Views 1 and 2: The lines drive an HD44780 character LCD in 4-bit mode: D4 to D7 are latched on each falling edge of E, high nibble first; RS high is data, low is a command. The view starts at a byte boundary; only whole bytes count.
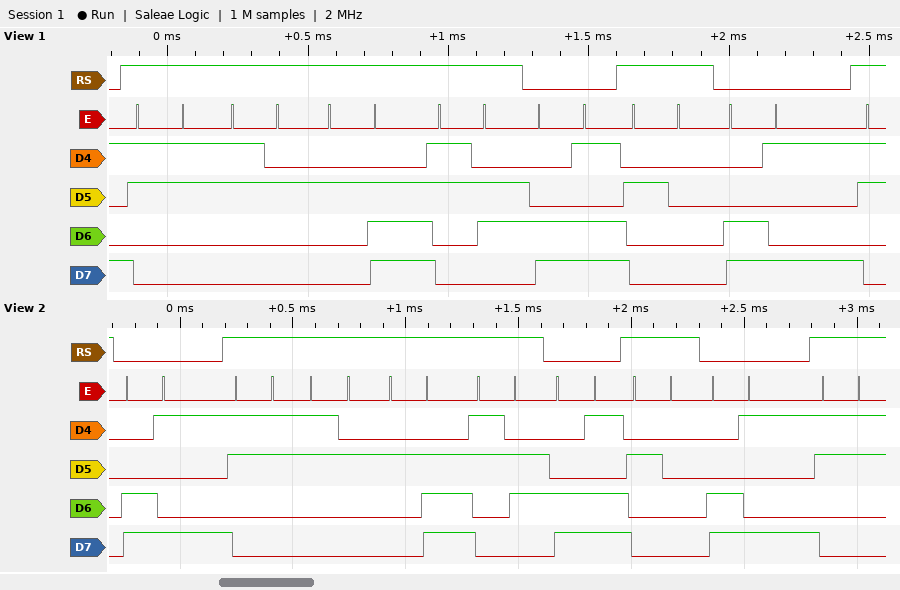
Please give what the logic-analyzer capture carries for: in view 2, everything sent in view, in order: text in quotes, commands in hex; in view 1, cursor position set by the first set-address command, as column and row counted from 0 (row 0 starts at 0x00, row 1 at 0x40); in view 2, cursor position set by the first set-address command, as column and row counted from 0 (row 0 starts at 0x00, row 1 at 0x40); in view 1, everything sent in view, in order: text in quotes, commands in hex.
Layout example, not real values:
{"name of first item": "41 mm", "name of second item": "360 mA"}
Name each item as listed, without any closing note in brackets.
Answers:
{"in view 2, everything sent in view, in order: text in quotes, commands in hex": "0xC9 \"32.6\" 0xCD \" \" 0xC9 \"3\"", "in view 1, cursor position set by the first set-address command, as column and row counted from 0": "column 13, row 1", "in view 2, cursor position set by the first set-address command, as column and row counted from 0": "column 9, row 1", "in view 1, everything sent in view, in order: text in quotes, commands in hex": "\"32.6\" 0xCD \" \" 0xC9"}
